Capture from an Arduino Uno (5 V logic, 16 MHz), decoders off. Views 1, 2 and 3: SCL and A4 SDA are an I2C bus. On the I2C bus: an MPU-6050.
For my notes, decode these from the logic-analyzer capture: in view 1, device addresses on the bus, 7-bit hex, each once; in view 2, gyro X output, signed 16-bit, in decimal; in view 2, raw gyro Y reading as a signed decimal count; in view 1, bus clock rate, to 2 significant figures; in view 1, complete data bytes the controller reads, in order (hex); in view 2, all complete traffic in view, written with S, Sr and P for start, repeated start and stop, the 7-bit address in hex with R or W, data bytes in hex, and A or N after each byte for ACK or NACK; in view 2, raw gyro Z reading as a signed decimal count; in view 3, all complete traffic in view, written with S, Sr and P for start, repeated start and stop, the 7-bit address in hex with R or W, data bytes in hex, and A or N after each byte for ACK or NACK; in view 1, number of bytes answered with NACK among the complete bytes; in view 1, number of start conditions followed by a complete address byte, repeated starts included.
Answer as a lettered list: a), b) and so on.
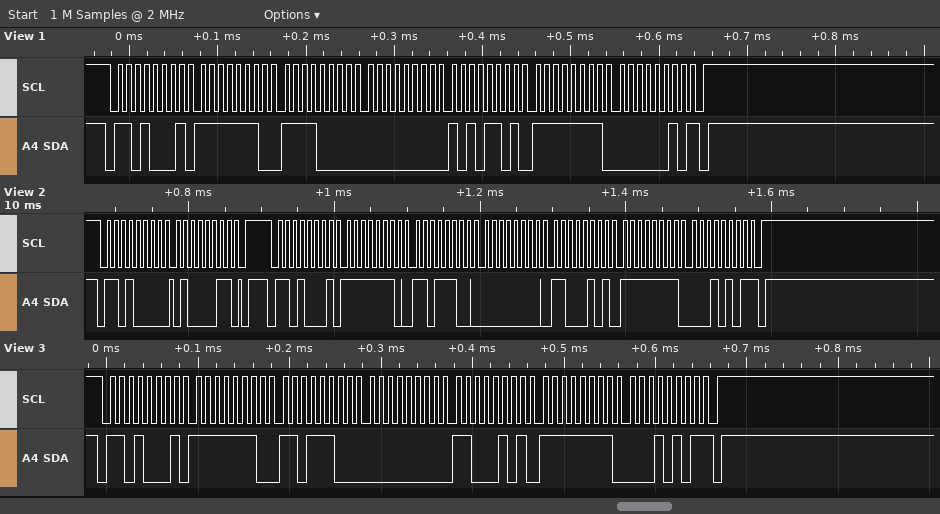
a) 0x68
b) -292
c) 197
d) 100 kHz
e) FE F0 00 AD FF 02
f) S 68W A 43 A P S 68R A FE A DC A 00 A C5 A FF A 15 N P
g) -235
h) S 68R A FE A DC A 00 A C5 A FF A 15 N P
i) 1
j) 1
